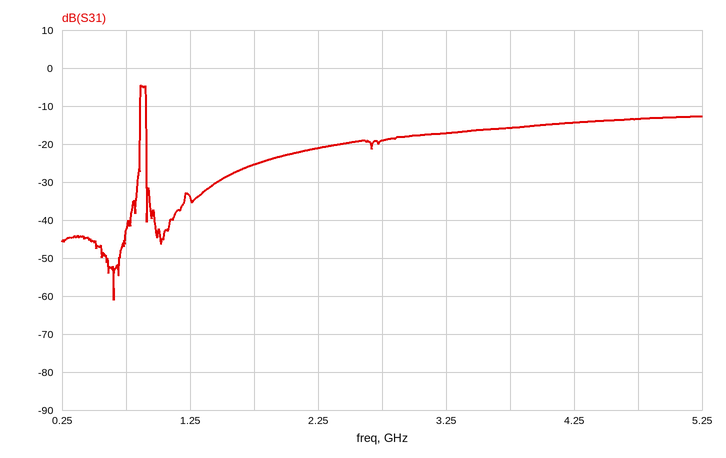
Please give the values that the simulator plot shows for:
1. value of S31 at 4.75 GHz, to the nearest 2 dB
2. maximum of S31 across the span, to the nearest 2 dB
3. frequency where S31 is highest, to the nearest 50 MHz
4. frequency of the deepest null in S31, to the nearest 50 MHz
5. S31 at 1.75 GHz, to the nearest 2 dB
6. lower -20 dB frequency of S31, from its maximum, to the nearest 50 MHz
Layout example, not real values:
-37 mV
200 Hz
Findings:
-14 dB
-4 dB
850 MHz
650 MHz
-26 dB
850 MHz
